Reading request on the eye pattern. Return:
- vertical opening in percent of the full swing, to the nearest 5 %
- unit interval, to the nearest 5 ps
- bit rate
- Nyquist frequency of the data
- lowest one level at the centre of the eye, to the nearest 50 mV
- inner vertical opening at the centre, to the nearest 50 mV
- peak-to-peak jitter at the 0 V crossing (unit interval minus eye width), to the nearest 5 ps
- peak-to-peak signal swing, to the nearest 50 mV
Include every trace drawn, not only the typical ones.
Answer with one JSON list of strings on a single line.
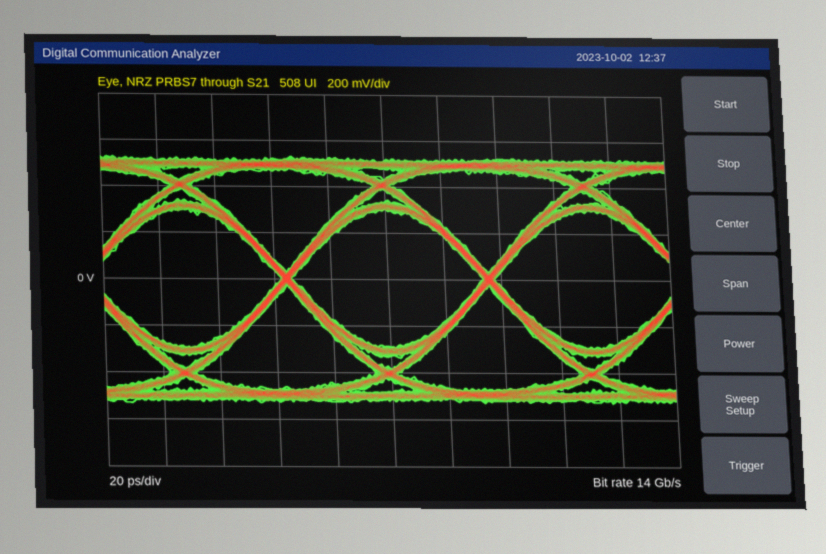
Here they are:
["55 %", "70 ps", "14 Gb/s", "7 GHz", "300 mV", "600 mV", "5 ps", "1.05 V"]
